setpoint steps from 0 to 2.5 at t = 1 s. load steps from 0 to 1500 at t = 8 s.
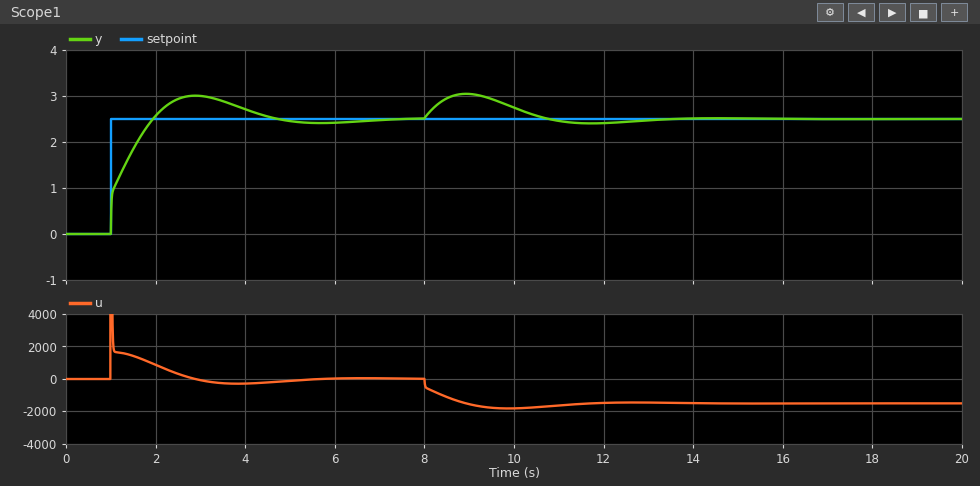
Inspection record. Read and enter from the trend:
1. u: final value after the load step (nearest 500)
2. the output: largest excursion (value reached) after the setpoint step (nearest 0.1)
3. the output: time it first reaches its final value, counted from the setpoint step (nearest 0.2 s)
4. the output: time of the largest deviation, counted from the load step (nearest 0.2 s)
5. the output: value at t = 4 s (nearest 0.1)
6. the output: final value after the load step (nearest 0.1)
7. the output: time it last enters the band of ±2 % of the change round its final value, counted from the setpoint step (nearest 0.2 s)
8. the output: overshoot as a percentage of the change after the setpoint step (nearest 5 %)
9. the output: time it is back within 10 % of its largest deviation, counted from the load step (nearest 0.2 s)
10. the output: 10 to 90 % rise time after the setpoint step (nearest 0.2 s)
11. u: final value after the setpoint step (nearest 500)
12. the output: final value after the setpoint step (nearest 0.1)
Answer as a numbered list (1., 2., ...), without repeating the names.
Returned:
1. -1500
2. 3.0
3. 1.0 s
4. 1.0 s
5. 2.7
6. 2.5
7. 5.6 s
8. 20 %
9. 4.6 s
10. 0.8 s
11. 0
12. 2.5
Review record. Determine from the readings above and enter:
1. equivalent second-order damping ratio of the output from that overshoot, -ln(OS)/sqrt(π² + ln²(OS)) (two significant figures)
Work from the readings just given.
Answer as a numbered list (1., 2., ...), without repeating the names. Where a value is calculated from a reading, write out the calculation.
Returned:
1. ln(0.2) = -1.609; 1.609 / sqrt(9.870 + 2.590) = 0.46
